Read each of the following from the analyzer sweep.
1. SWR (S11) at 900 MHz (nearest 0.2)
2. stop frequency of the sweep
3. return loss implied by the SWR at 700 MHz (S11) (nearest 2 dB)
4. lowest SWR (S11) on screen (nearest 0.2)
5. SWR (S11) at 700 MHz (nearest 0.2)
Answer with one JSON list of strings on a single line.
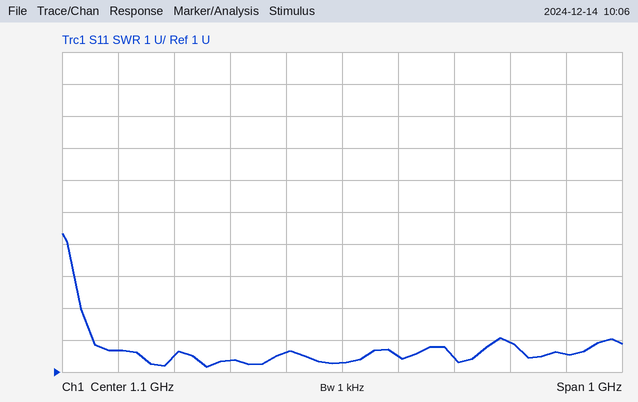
["1.4", "1.6 GHz", "12 dB", "1.2", "1.6"]
